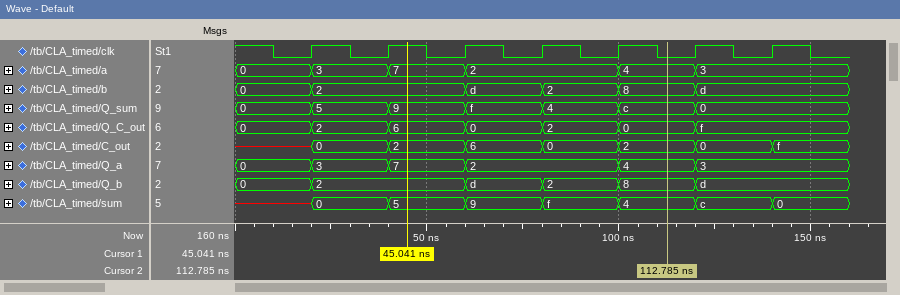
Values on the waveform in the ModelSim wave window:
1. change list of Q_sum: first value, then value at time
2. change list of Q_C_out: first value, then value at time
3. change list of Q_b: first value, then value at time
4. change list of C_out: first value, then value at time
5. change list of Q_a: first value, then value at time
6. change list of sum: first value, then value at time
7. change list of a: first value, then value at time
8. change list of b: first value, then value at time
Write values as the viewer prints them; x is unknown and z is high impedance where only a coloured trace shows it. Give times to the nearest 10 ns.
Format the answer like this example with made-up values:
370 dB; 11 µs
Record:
0, 5 at 20 ns, 9 at 40 ns, f at 60 ns, 4 at 80 ns, c at 100 ns, 0 at 120 ns; 0, 2 at 20 ns, 6 at 40 ns, 0 at 60 ns, 2 at 80 ns, 0 at 100 ns, f at 120 ns; 0, 2 at 20 ns, d at 60 ns, 2 at 80 ns, 8 at 100 ns, d at 120 ns; x, 0 at 20 ns, 2 at 40 ns, 6 at 60 ns, 0 at 80 ns, 2 at 100 ns, 0 at 120 ns, f at 140 ns; 0, 3 at 20 ns, 7 at 40 ns, 2 at 60 ns, 4 at 100 ns, 3 at 120 ns; x, 0 at 20 ns, 5 at 40 ns, 9 at 60 ns, f at 80 ns, 4 at 100 ns, c at 120 ns, 0 at 140 ns; 0, 3 at 20 ns, 7 at 40 ns, 2 at 60 ns, 4 at 100 ns, 3 at 120 ns; 0, 2 at 20 ns, d at 60 ns, 2 at 80 ns, 8 at 100 ns, d at 120 ns
